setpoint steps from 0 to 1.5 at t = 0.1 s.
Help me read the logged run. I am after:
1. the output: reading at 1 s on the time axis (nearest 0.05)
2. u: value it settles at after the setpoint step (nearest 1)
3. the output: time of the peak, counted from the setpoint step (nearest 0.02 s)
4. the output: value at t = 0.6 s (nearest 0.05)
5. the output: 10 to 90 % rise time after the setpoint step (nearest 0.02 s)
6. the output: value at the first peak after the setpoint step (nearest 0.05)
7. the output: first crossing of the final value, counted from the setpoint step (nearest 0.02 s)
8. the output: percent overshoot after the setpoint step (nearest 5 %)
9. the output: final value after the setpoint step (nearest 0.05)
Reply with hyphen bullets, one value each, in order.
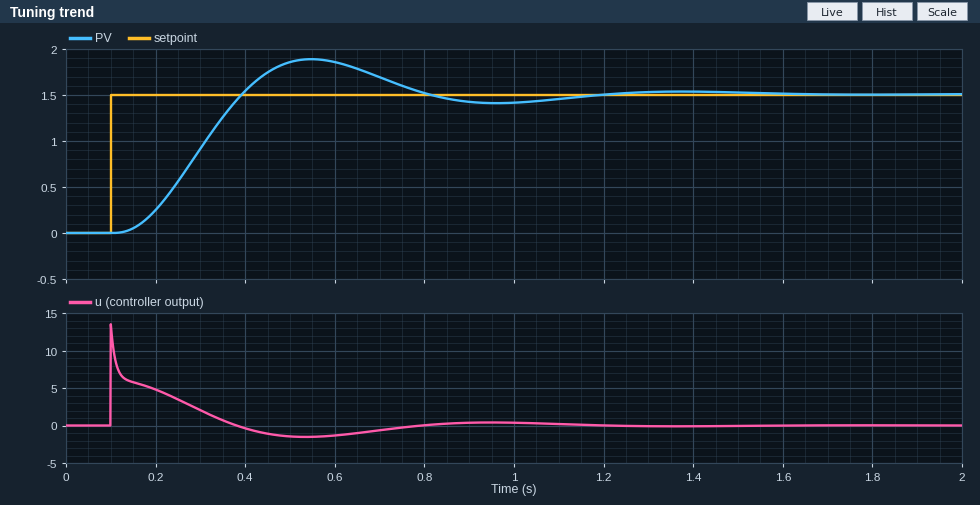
- 1.40
- 0
- 0.44 s
- 1.85
- 0.18 s
- 1.90
- 0.30 s
- 25 %
- 1.50
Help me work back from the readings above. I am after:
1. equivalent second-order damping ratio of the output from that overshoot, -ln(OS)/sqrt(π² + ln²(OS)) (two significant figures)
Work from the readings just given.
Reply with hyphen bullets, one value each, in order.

- 0.40
